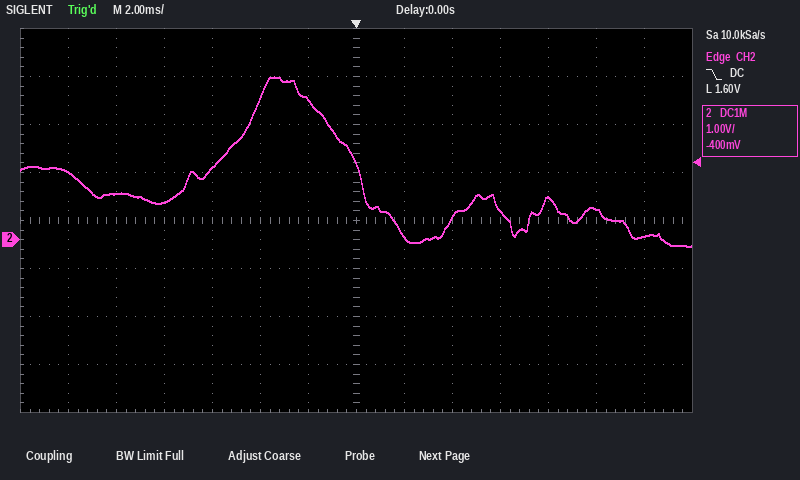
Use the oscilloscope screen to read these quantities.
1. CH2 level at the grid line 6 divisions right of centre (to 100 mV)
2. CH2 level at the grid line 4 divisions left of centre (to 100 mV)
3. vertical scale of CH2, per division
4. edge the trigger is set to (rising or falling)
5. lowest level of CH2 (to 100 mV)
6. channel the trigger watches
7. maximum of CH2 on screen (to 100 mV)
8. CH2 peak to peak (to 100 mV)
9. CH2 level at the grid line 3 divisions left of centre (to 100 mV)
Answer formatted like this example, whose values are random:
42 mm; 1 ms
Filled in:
100 mV; 800 mV; 1 V; falling; -100 mV; CH2; 3.4 V; 3.5 V; 1.5 V
